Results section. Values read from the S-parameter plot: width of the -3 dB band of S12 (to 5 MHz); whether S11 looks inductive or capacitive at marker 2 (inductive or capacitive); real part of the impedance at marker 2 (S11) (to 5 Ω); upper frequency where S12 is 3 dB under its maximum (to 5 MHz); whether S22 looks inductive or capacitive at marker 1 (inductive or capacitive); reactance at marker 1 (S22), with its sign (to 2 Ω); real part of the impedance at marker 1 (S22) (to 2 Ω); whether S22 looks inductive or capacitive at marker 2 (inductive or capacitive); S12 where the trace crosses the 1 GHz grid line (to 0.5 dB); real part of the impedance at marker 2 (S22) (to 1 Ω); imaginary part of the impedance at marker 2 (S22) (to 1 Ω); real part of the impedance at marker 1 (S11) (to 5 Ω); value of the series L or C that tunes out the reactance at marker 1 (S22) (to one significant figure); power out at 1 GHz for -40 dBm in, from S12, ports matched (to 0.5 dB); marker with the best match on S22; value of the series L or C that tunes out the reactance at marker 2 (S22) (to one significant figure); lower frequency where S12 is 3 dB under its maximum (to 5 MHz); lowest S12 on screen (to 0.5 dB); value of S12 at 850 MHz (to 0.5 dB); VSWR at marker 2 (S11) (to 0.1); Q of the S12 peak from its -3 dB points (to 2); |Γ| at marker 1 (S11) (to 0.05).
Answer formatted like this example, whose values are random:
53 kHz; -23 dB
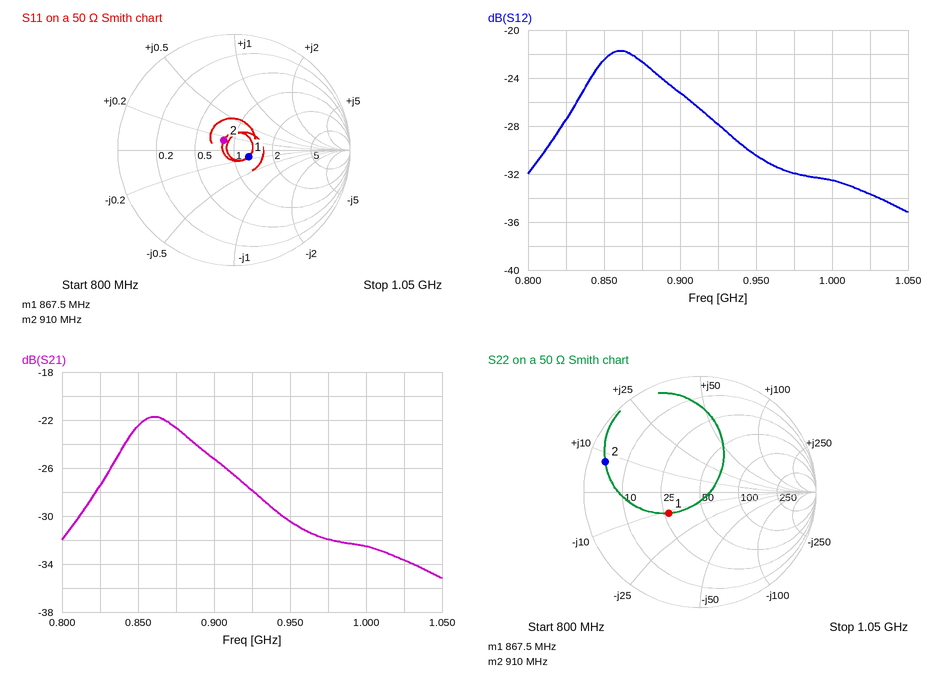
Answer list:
55 MHz; inductive; 40 Ω; 895 MHz; capacitive; -12 Ω; 28 Ω; inductive; -32.5 dB; 4 Ω; +8 Ω; 65 Ω; 2 nH; -72.5 dBm; marker 1; 20 pF; 840 MHz; -35.0 dB; -22.5 dB; 1.3; 16; 0.15
